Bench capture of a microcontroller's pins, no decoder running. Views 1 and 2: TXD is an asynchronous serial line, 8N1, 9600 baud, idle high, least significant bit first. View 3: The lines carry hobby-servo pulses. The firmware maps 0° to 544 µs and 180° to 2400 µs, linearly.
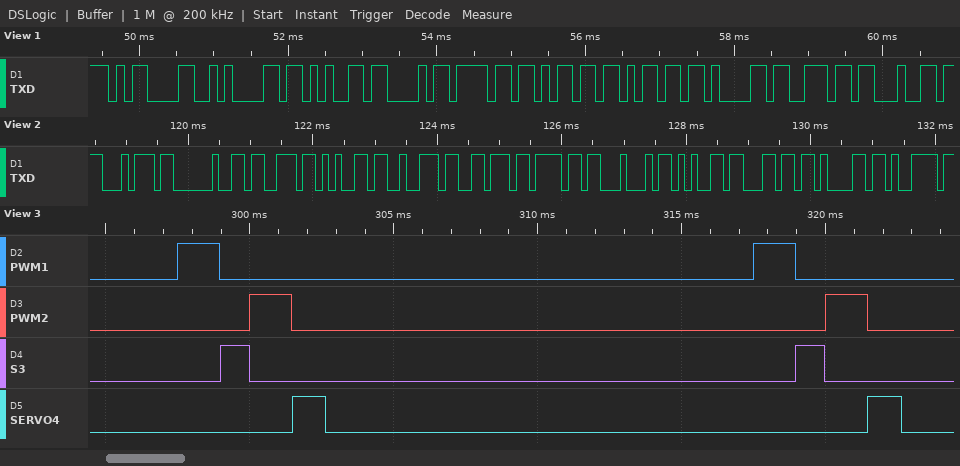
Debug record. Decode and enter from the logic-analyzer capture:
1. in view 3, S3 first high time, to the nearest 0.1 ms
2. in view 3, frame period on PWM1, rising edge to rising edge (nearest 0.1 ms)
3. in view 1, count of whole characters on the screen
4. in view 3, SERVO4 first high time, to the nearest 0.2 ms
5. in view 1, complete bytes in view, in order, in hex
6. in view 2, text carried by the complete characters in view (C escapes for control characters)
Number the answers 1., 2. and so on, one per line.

1. 1.0 ms
2. 20.0 ms
3. 10
4. 1.2 ms
5. 0D 0A 2B 43 6F 6D 6D 61 6E 64
6. "t servoDelay"
